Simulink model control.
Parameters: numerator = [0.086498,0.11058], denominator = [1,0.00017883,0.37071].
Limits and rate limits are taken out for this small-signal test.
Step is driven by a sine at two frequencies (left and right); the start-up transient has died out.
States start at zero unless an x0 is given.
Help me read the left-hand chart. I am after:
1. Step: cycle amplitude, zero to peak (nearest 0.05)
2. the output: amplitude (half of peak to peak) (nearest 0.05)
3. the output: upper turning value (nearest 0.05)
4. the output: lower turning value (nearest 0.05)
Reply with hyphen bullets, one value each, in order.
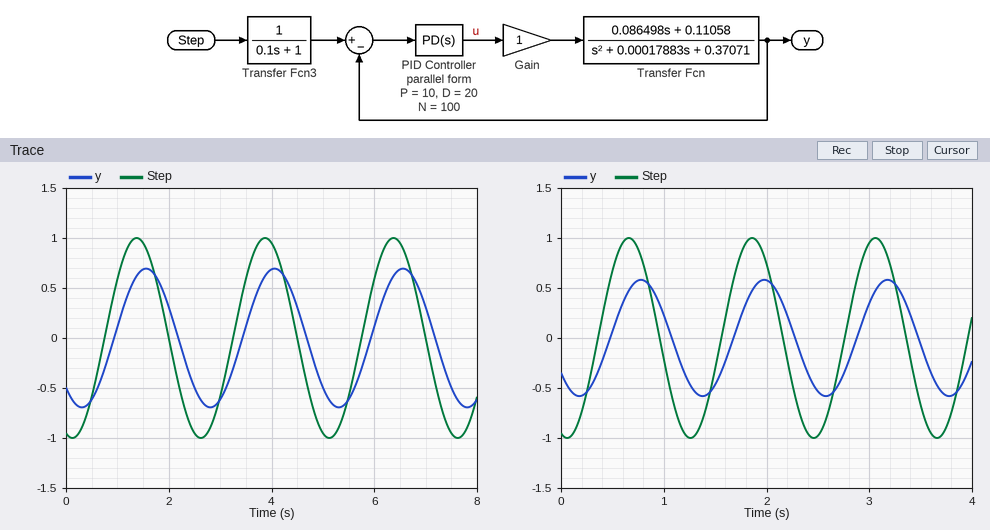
- 1.00
- 0.70
- 0.70
- -0.70
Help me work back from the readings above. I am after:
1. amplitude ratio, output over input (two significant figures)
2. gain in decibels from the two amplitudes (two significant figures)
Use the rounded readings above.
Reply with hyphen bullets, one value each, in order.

- 0.70
- -3.1 dB
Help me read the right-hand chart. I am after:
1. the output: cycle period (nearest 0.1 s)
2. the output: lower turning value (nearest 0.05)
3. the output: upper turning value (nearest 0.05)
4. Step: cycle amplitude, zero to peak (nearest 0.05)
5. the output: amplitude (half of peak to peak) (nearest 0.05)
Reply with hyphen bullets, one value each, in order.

- 1.2 s
- -0.60
- 0.60
- 1.00
- 0.60
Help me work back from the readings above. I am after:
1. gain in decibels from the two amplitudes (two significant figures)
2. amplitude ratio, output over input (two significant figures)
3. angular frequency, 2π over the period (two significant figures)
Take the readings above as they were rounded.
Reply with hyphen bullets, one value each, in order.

- -4.4 dB
- 0.60
- 5.2 rad/s
